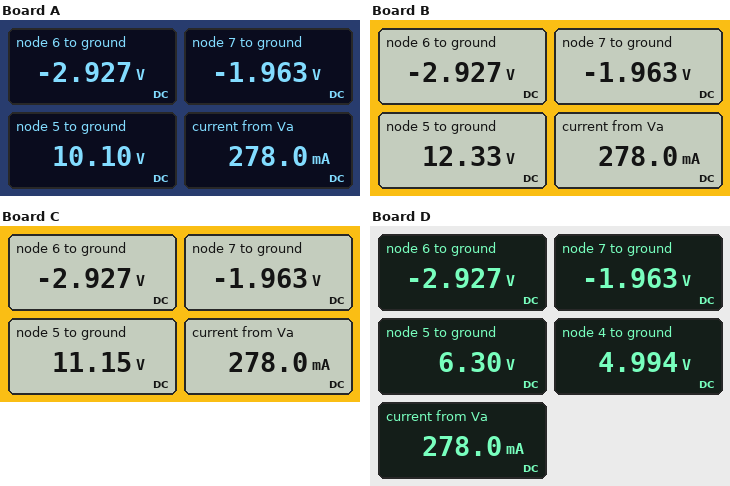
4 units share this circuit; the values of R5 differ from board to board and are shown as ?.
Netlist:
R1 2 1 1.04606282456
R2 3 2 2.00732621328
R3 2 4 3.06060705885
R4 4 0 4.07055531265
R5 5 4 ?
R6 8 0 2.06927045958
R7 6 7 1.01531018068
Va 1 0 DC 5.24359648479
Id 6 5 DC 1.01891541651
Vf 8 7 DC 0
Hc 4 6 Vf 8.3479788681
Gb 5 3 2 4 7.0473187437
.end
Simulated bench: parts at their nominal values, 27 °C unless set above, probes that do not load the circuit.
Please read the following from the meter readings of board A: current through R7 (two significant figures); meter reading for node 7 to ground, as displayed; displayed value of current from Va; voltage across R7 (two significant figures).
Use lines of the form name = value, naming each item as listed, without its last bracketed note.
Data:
current through R7 = 950 mA
meter reading for node 7 to ground, as displayed = -1.963 V
displayed value of current from Va = 278.0 mA
voltage across R7 = 960 mV
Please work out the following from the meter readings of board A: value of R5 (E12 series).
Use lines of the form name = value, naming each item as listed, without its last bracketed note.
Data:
value of R5 = 3.9 Ω
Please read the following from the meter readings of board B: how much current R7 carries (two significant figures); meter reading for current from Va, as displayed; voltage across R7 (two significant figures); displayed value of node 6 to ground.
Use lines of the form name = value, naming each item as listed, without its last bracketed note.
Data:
how much current R7 carries = 950 mA
meter reading for current from Va, as displayed = 278.0 mA
voltage across R7 = 960 mV
displayed value of node 6 to ground = -2.927 V
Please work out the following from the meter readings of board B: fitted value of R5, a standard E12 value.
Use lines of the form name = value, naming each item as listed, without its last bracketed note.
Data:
fitted value of R5, a standard E12 value = 5.6 Ω
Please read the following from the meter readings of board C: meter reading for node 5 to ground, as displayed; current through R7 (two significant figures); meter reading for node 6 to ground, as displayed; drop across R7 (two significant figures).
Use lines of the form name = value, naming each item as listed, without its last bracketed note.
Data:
meter reading for node 5 to ground, as displayed = 11.15 V
current through R7 = 950 mA
meter reading for node 6 to ground, as displayed = -2.927 V
drop across R7 = 960 mV
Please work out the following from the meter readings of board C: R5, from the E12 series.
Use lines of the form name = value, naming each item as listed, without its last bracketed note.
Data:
R5, from the E12 series = 4.7 Ω
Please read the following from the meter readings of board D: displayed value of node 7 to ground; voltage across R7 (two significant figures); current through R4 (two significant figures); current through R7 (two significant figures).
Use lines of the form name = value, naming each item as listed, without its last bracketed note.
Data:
displayed value of node 7 to ground = -1.963 V
voltage across R7 = 960 mV
current through R4 = 1.2 A
current through R7 = 950 mA
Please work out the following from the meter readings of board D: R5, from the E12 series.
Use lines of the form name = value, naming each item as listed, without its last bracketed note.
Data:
R5, from the E12 series = 1 Ω
